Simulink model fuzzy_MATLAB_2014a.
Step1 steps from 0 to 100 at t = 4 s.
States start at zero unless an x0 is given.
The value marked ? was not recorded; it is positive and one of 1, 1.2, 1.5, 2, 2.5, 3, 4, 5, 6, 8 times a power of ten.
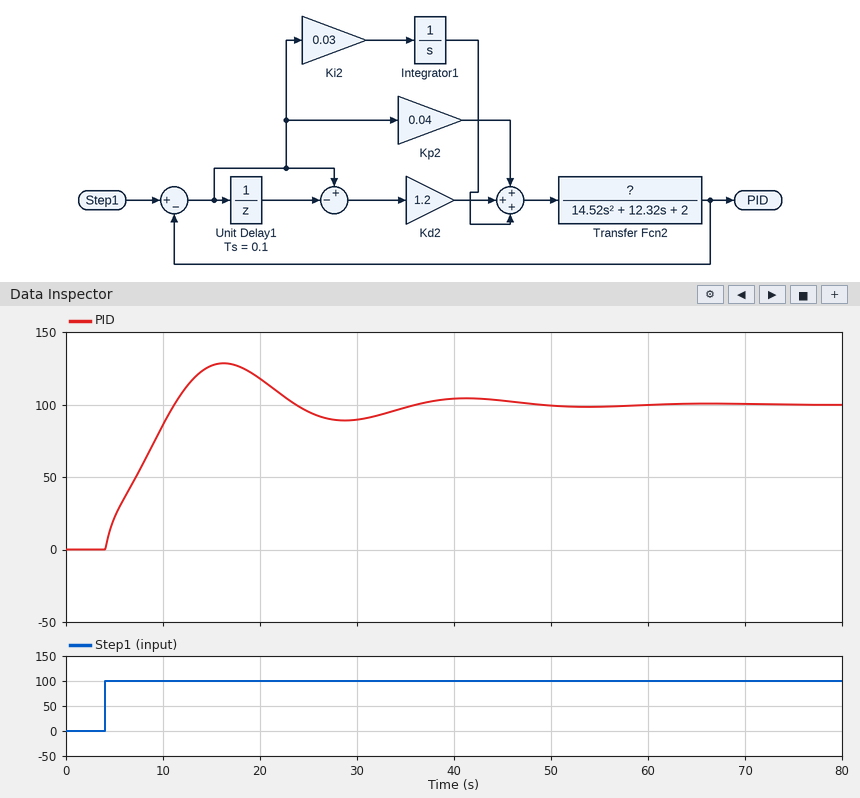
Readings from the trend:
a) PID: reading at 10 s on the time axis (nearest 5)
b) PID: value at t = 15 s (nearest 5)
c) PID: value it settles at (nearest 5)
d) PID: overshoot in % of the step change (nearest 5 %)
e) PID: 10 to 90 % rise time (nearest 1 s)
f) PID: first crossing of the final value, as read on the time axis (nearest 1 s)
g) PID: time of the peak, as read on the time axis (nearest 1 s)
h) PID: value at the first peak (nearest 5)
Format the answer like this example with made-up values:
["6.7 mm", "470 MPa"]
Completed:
["85", "125", "100", "30 %", "6 s", "11 s", "16 s", "130"]
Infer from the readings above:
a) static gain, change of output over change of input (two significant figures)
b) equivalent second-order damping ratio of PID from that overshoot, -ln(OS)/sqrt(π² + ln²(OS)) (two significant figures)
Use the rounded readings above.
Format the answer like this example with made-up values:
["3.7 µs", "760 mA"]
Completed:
["1.0", "0.36"]
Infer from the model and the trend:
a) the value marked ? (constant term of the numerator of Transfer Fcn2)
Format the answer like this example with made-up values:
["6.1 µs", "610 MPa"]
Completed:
["40"]
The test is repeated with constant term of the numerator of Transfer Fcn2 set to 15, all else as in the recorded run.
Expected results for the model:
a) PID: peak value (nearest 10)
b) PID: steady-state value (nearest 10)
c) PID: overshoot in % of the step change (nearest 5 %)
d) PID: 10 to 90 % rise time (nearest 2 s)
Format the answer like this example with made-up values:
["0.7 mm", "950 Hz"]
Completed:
["120", "100", "20 %", "10 s"]
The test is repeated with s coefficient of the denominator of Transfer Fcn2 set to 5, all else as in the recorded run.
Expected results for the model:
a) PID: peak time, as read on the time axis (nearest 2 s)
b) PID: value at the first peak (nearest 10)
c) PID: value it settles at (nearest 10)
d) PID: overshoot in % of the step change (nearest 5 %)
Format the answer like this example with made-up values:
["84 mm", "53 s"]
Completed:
["14 s", "120", "100", "20 %"]
